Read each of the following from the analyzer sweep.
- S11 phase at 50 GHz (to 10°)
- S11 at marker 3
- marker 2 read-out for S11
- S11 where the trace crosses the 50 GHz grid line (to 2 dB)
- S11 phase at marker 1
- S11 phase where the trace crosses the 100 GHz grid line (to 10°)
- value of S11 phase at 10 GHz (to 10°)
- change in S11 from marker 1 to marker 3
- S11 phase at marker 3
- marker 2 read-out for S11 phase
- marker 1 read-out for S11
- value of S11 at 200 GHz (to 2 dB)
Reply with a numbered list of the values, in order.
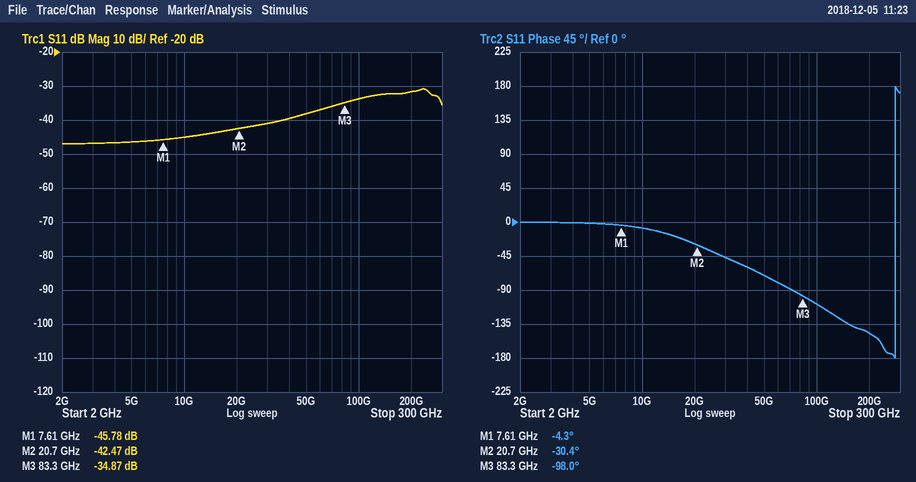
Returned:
1. -70°
2. -34.87 dB
3. -42.47 dB
4. -38 dB
5. -4.3°
6. -110°
7. -10°
8. 10.91 dB
9. -98.0°
10. -30.4°
11. -45.78 dB
12. -32 dB
